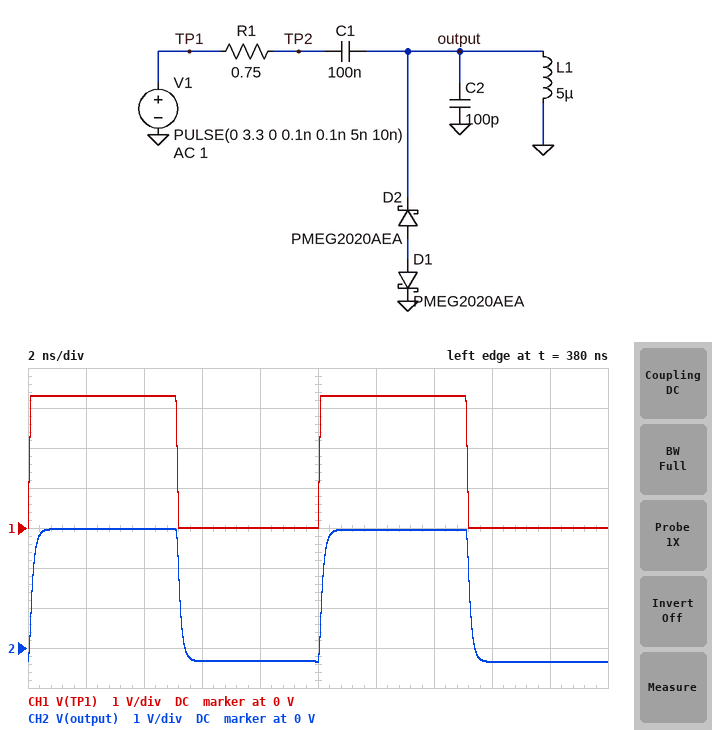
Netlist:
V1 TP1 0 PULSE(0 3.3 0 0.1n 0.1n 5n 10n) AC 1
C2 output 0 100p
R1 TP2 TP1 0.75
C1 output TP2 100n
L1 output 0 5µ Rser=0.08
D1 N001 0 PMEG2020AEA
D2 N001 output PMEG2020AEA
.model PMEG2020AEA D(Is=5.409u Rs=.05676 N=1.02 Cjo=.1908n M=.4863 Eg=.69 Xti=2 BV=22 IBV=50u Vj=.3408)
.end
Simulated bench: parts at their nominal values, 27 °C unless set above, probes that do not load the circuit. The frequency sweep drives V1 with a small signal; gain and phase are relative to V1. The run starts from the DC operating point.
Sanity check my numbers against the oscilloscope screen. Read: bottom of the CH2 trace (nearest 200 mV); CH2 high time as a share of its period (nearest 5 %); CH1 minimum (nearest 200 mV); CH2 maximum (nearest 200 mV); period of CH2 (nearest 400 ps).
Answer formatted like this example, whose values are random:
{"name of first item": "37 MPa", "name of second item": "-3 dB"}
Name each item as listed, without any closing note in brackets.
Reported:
{"bottom of the CH2 trace": "-400 mV", "CH2 high time as a share of its period": "50 %", "CH1 minimum": "0 V", "CH2 maximum": "3.0 V", "period of CH2": "10.0 ns"}
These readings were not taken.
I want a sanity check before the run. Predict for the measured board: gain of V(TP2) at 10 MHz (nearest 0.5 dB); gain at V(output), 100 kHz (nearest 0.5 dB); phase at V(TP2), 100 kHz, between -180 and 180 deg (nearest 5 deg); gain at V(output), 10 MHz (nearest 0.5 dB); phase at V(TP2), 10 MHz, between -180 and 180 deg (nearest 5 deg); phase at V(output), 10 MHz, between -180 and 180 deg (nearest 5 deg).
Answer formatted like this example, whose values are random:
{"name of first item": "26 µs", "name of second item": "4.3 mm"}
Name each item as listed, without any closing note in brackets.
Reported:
{"gain of V(TP2) at 10 MHz": "0 dB", "gain at V(output), 100 kHz": "-12.0 dB", "phase at V(TP2), 100 kHz, between -180 and 180 deg": "-5 deg", "gain at V(output), 10 MHz": "0 dB", "phase at V(TP2), 10 MHz, between -180 and 180 deg": "0 deg", "phase at V(output), 10 MHz, between -180 and 180 deg": "0 deg"}
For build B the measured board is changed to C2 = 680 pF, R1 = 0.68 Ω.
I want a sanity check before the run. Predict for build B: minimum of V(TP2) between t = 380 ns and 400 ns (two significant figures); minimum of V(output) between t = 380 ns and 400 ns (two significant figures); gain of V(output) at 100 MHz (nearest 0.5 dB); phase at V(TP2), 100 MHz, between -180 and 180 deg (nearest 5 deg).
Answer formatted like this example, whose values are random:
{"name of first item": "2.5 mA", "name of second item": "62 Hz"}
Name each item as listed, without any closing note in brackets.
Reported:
{"minimum of V(TP2) between t = 380 ns and 400 ns": "-83 mV", "minimum of V(output) between t = 380 ns and 400 ns": "-340 mV", "gain of V(output) at 100 MHz": "-0.5 dB", "phase at V(TP2), 100 MHz, between -180 and 180 deg": "-20 deg"}
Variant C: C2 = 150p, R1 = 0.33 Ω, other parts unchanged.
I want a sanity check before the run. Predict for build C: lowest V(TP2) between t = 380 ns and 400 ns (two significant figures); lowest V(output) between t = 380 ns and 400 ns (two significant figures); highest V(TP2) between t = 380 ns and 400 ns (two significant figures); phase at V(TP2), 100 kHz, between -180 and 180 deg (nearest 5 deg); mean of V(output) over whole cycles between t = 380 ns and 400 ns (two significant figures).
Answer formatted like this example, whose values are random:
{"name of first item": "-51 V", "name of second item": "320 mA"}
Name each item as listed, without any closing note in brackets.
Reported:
{"lowest V(TP2) between t = 380 ns and 400 ns": "-41 mV", "lowest V(output) between t = 380 ns and 400 ns": "-300 mV", "highest V(TP2) between t = 380 ns and 400 ns": "3.3 V", "phase at V(TP2), 100 kHz, between -180 and 180 deg": "0 deg", "mean of V(output) over whole cycles between t = 380 ns and 400 ns": "1.4 V"}
